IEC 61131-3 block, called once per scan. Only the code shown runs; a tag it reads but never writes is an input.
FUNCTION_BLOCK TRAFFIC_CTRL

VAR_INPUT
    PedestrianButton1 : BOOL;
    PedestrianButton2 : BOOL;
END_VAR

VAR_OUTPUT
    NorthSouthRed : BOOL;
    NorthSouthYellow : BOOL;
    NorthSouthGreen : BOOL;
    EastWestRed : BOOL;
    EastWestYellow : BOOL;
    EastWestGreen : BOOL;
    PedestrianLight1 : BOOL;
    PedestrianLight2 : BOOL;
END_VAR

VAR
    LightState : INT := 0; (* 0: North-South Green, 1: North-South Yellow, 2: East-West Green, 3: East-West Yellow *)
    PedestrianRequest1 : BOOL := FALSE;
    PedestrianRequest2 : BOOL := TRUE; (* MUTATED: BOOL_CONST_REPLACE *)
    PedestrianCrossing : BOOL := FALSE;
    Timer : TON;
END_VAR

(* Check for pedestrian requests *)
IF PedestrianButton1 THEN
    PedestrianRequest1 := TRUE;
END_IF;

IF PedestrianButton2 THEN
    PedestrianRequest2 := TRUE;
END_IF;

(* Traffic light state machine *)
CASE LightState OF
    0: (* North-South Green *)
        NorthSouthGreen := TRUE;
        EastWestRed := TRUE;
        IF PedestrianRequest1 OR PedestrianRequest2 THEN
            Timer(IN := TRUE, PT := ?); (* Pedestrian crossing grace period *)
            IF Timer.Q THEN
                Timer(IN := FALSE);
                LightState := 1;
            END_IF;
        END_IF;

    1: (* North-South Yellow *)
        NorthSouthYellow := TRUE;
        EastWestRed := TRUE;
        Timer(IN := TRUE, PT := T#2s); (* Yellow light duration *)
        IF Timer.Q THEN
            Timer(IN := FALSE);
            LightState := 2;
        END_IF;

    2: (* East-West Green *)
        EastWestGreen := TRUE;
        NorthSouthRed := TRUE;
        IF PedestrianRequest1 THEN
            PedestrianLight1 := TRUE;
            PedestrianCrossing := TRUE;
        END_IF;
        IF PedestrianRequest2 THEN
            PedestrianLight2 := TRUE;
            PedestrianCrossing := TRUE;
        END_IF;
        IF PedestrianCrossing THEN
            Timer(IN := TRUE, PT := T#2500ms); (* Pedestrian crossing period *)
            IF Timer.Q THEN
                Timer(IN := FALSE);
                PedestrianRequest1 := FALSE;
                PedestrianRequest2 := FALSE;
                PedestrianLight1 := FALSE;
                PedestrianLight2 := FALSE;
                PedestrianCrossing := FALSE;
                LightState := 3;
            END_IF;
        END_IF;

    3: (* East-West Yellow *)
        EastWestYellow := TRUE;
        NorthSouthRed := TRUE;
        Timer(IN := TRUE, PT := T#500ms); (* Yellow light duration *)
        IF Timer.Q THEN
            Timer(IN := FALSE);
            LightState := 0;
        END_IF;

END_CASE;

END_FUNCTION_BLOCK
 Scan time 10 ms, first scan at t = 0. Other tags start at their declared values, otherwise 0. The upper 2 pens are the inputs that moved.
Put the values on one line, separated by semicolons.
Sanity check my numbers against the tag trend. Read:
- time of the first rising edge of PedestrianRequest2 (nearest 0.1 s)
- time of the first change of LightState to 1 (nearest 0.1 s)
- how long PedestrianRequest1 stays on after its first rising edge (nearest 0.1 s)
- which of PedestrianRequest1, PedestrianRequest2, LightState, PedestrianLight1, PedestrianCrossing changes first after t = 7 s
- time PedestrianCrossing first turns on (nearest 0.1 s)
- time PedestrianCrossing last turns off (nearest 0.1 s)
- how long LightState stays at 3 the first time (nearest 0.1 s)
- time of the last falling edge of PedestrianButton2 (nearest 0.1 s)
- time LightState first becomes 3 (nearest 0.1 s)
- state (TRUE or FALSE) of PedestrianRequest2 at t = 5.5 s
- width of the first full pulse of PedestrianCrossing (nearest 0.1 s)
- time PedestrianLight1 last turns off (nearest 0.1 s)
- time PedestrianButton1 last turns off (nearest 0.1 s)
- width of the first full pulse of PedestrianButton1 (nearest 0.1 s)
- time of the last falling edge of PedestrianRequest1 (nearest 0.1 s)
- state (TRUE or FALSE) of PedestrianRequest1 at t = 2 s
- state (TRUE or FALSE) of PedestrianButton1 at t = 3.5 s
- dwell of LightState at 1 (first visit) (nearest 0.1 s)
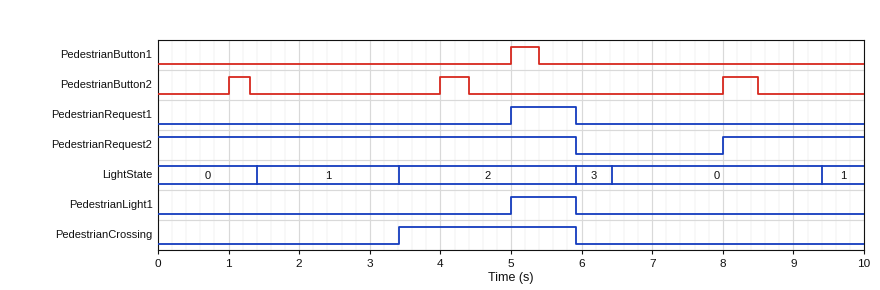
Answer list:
8.0 s; 1.4 s; 0.9 s; PedestrianRequest2; 3.4 s; 5.9 s; 0.5 s; 8.5 s; 5.9 s; TRUE; 2.5 s; 5.9 s; 5.4 s; 0.4 s; 5.9 s; FALSE; FALSE; 2.0 s
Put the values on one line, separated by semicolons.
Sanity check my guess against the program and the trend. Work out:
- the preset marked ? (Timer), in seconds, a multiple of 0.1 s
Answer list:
1.4 s
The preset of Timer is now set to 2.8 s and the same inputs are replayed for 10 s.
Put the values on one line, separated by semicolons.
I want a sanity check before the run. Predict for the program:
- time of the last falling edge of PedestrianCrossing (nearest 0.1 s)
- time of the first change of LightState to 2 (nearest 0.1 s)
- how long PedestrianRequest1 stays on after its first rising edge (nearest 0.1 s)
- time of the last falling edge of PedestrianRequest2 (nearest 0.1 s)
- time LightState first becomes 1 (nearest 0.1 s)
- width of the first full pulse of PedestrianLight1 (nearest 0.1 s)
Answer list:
7.3 s; 4.8 s; 2.3 s; 7.3 s; 2.8 s; 2.3 s
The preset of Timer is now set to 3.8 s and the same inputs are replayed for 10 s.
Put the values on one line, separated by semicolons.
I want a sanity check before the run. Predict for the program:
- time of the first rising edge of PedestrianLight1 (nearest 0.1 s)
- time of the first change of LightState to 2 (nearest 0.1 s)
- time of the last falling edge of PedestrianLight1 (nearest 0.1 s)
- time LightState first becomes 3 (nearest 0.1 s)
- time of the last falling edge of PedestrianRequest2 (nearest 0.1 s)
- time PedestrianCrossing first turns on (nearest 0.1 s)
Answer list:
5.8 s; 5.8 s; 8.3 s; 8.3 s; 8.3 s; 5.8 s
